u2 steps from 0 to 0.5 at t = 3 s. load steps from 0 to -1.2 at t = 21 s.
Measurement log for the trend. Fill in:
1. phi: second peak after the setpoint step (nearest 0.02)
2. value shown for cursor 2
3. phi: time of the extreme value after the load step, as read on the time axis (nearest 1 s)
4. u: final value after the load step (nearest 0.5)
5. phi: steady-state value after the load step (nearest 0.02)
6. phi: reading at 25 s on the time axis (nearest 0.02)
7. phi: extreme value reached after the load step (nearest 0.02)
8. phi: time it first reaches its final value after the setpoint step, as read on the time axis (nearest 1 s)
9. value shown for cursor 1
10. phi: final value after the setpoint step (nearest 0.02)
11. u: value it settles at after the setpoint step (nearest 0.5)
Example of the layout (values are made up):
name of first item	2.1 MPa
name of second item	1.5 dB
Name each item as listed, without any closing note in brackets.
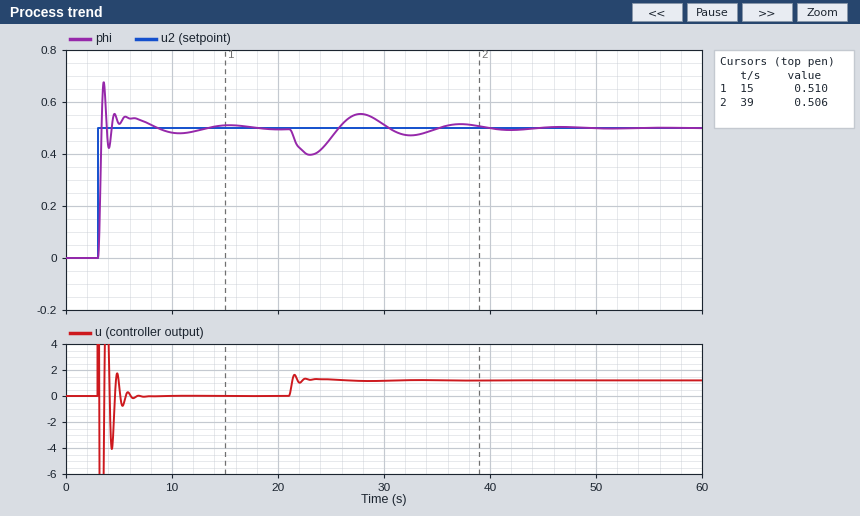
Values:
phi: second peak after the setpoint step	0.56
value shown for cursor 2	0.506
phi: time of the extreme value after the load step, as read on the time axis	23 s
u: final value after the load step	1.0
phi: steady-state value after the load step	0.50
phi: reading at 25 s on the time axis	0.46
phi: extreme value reached after the load step	0.40
phi: time it first reaches its final value after the setpoint step, as read on the time axis	3 s
value shown for cursor 1	0.510
phi: final value after the setpoint step	0.50
u: value it settles at after the setpoint step	0.0
